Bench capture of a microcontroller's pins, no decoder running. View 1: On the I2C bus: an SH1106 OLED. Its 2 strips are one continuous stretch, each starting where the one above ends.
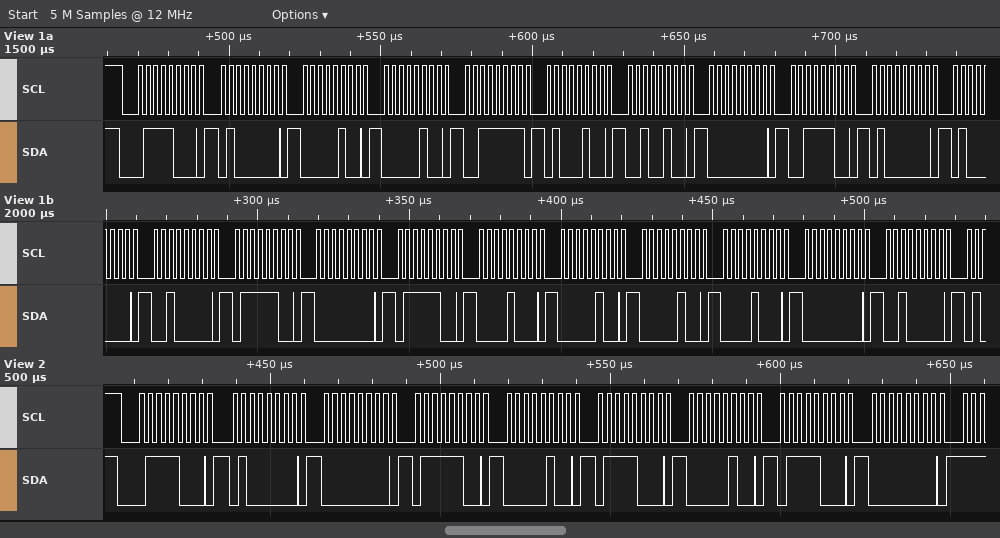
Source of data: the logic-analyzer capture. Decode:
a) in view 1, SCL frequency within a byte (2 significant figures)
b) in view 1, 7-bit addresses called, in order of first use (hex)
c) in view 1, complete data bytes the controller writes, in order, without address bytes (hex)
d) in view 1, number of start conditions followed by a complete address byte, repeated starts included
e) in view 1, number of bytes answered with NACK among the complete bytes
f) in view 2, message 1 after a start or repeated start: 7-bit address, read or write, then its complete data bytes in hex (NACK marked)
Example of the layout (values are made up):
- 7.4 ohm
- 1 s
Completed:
- 400 kHz
- 0x3C
- 40 04 04 3F 44 24 00 3C 40 40 20 7C 00 7C 08 04 04 08 00 20
- 1
- 0
- 0x3C write: 40 00 7C 04 78 04 78 00
